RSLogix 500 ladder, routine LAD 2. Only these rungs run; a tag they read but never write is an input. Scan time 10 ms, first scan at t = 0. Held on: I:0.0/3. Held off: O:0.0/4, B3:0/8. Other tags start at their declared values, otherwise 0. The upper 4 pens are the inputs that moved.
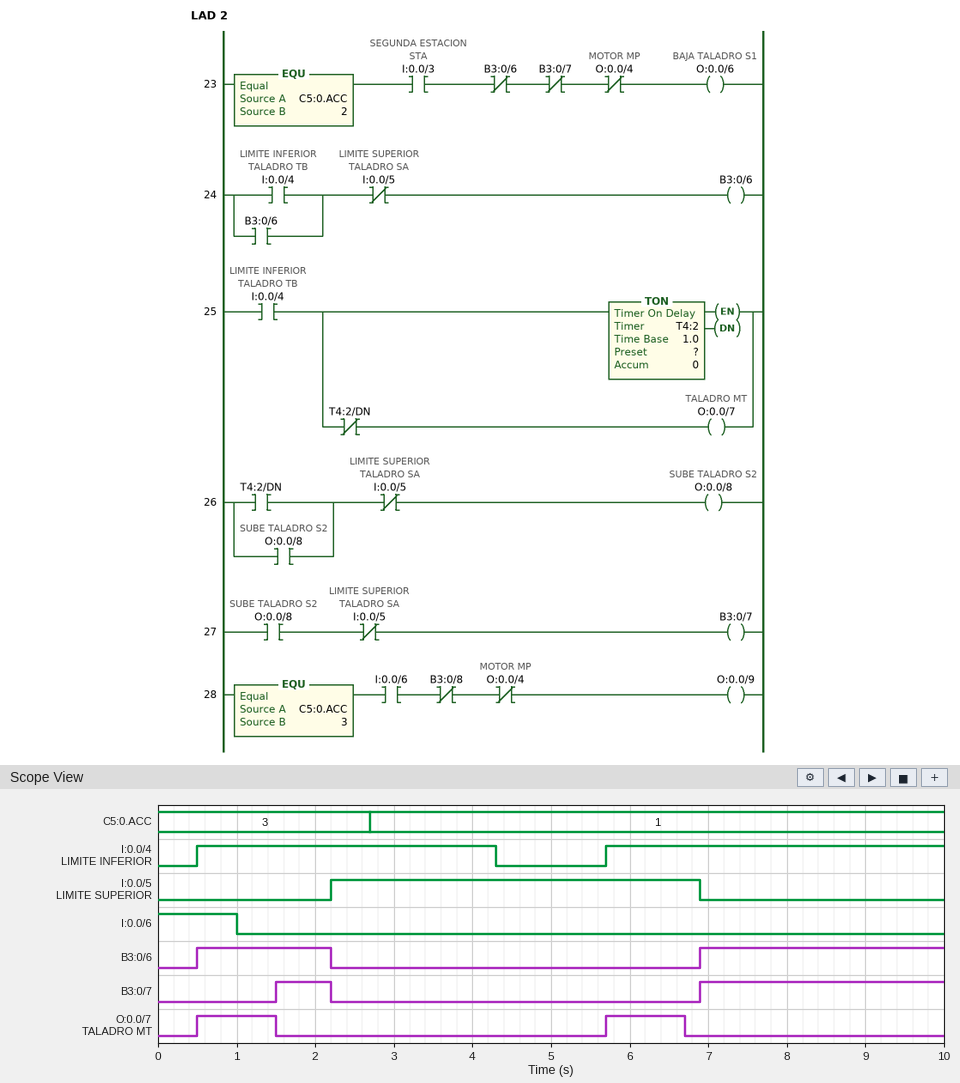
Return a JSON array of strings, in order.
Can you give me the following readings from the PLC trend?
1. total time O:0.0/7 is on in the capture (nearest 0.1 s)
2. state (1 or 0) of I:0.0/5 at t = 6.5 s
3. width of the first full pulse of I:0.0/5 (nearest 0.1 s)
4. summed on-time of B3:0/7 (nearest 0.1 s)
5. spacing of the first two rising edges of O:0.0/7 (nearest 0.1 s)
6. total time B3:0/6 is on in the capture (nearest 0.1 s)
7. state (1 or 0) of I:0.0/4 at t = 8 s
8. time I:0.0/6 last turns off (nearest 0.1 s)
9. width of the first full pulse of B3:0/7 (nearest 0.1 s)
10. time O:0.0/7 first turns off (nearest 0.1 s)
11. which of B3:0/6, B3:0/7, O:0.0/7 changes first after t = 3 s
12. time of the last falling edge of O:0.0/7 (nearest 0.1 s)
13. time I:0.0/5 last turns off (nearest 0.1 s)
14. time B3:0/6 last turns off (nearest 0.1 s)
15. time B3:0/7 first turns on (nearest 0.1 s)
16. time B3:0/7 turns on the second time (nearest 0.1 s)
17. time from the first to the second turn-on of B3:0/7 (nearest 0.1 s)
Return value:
["2.0 s", "1", "4.7 s", "3.8 s", "5.2 s", "4.8 s", "1", "1.0 s", "0.7 s", "1.5 s", "O:0.0/7", "6.7 s", "6.9 s", "2.2 s", "1.5 s", "6.9 s", "5.4 s"]
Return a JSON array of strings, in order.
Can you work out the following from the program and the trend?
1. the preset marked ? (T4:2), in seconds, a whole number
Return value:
["1 s"]
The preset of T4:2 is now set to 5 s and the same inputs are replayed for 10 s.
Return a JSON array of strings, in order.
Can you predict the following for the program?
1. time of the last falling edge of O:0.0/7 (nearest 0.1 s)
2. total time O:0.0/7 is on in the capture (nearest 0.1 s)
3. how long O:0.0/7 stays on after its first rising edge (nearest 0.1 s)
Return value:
["4.3 s", "8.1 s", "3.8 s"]
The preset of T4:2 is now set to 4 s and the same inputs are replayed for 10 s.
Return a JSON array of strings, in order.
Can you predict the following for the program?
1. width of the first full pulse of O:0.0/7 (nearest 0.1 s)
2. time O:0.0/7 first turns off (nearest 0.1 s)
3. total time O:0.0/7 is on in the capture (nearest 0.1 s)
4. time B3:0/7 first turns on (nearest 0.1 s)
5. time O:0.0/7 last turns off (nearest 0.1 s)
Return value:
["3.8 s", "4.3 s", "7.8 s", "9.7 s", "9.7 s"]
